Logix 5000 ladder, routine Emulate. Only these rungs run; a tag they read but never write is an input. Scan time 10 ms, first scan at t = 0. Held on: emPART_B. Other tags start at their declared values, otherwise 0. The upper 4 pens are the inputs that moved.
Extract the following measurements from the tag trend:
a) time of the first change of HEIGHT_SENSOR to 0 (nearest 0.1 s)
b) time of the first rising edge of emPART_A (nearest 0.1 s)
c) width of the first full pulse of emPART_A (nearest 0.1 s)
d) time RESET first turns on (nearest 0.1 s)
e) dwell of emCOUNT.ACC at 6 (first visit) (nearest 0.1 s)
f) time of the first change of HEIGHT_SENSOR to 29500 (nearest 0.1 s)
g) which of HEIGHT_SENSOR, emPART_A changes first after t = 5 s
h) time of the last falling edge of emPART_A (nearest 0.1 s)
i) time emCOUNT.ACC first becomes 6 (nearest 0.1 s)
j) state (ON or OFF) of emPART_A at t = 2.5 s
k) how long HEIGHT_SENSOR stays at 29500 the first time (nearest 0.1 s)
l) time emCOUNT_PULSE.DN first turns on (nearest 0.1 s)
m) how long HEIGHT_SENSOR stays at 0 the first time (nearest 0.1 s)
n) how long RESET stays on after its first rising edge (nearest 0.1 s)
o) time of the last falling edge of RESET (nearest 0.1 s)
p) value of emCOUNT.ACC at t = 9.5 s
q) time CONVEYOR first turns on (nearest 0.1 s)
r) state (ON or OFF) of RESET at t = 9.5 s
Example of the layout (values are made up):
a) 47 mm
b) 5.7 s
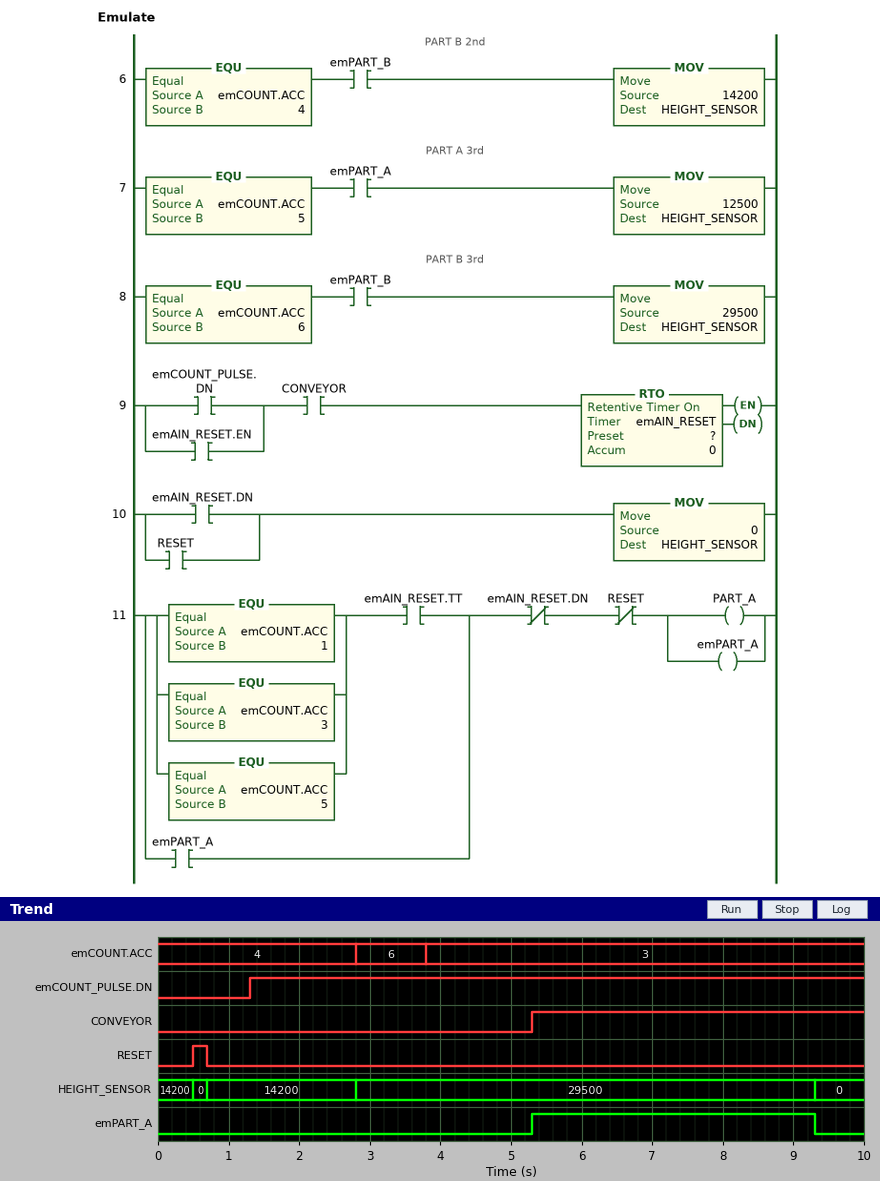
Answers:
a) 0.5 s
b) 5.3 s
c) 4.0 s
d) 0.5 s
e) 1.0 s
f) 2.8 s
g) emPART_A
h) 9.3 s
i) 2.8 s
j) OFF
k) 6.5 s
l) 1.3 s
m) 0.2 s
n) 0.2 s
o) 0.7 s
p) 3
q) 5.3 s
r) OFF
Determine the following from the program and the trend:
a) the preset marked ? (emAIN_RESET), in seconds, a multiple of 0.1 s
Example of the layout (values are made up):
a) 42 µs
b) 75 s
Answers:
a) 4.0 s
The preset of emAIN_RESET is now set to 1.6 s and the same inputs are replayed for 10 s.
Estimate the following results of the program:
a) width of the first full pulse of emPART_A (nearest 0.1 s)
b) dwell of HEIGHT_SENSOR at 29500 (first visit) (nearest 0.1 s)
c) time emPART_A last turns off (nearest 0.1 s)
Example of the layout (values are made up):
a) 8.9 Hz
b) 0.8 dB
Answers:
a) 1.6 s
b) 4.1 s
c) 6.9 s
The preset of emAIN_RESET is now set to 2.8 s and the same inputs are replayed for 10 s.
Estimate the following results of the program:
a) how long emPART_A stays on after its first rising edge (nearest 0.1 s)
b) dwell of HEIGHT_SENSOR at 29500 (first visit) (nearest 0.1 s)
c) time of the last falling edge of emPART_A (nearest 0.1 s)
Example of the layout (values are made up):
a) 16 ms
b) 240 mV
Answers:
a) 2.8 s
b) 5.3 s
c) 8.1 s
